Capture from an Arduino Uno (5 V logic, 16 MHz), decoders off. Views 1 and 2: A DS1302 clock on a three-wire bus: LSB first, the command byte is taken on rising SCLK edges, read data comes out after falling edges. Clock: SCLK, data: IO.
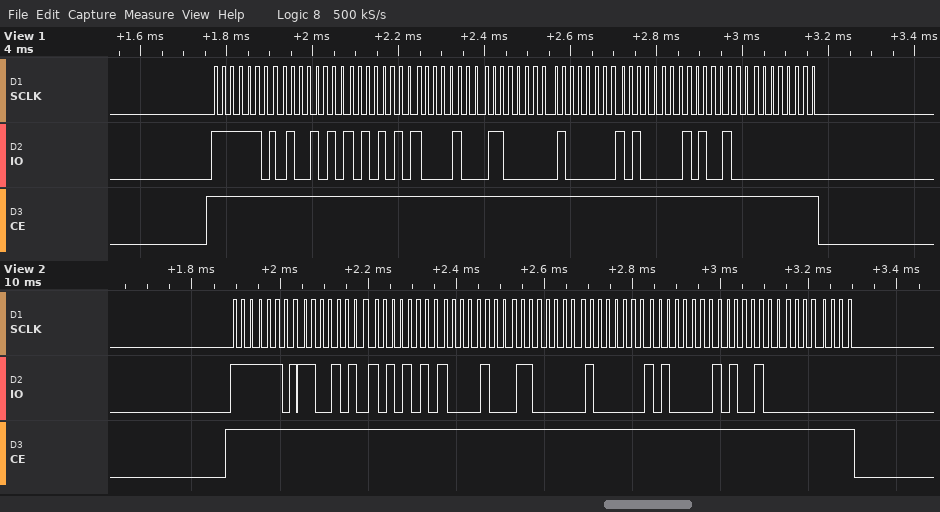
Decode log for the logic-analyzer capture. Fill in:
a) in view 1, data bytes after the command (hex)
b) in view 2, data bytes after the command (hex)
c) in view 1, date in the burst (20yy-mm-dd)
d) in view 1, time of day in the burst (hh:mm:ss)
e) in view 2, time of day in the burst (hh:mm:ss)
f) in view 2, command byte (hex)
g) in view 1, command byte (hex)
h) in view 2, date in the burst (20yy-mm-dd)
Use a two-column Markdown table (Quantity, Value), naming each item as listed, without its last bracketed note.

| Quantity | Value |
|---|---|
| in view 1, data bytes after the command | 52 55 21 06 02 05 25 00 |
| in view 2, data bytes after the command | 53 55 21 06 02 05 25 00 |
| in view 1, date in the burst | 2025-02-06 |
| in view 1, time of day in the burst | 21:55:52 |
| in view 2, time of day in the burst | 21:55:53 |
| in view 2, command byte | 0xBF |
| in view 1, command byte | 0xBF |
| in view 2, date in the burst | 2025-02-06 |
